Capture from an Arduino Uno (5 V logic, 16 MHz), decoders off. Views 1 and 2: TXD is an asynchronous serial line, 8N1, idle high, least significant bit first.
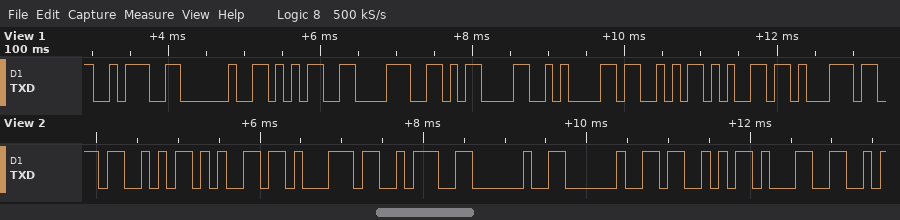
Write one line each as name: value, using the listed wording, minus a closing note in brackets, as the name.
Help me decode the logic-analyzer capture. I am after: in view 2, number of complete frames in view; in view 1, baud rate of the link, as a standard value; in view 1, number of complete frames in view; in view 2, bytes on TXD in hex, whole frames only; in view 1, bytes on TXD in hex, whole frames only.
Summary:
in view 2, number of complete frames in view: 8
in view 1, baud rate of the link, as a standard value: 9600 baud
in view 1, number of complete frames in view: 9
in view 2, bytes on TXD in hex, whole frames only: 0x53 0x65 0x71 0x3A 0x20 0x20 0x53 0x31
in view 1, bytes on TXD in hex, whole frames only: 3A 20 35 38 0D 0A 53 65 71
